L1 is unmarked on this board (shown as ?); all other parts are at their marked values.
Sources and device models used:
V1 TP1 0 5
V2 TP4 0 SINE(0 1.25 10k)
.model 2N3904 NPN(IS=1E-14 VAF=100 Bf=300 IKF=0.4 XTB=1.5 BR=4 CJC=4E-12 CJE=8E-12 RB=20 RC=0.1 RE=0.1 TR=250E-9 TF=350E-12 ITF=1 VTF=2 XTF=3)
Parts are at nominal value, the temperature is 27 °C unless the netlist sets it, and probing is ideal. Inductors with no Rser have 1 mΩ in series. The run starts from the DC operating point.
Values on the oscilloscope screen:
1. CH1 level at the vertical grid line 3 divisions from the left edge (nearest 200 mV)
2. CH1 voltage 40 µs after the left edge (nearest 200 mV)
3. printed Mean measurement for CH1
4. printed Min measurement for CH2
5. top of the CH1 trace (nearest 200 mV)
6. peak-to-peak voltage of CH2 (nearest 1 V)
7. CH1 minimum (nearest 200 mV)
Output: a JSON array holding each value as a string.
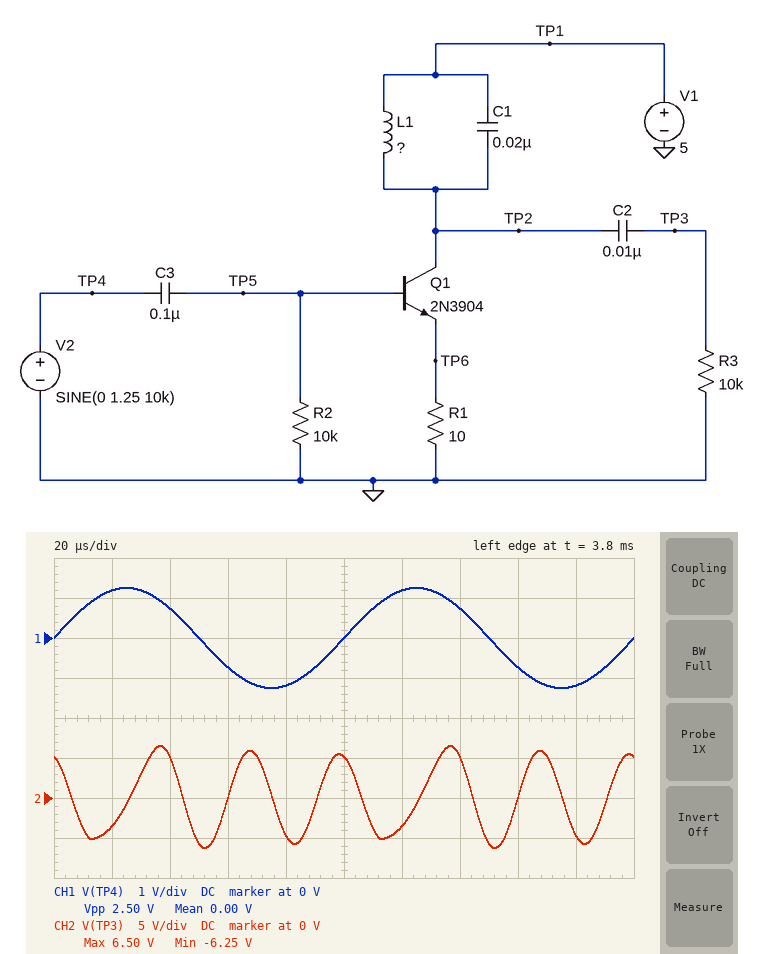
["-800 mV", "800 mV", "0.00 V", "-6.25 V", "1.2 V", "13 V", "-1.2 V"]
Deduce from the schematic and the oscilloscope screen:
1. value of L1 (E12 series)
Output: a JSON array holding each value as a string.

["1.2 mH"]
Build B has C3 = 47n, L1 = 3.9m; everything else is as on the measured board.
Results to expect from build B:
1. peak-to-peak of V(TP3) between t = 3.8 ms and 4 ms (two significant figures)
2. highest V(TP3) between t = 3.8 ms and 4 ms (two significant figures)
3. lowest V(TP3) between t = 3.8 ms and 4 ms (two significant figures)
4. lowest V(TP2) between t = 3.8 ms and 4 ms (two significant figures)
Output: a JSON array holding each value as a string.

["9.8 V", "4.7 V", "-5.1 V", "9.6 mV"]
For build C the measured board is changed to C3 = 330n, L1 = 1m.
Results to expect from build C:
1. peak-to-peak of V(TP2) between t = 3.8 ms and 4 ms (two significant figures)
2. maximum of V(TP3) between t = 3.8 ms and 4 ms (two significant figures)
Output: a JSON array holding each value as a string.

["11 V", "5.7 V"]
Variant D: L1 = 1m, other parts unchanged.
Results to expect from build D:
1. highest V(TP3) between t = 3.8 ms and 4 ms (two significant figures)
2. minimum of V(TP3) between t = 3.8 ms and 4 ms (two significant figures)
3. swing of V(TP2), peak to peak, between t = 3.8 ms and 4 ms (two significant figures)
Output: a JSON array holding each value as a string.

["5.7 V", "-5.6 V", "11 V"]
